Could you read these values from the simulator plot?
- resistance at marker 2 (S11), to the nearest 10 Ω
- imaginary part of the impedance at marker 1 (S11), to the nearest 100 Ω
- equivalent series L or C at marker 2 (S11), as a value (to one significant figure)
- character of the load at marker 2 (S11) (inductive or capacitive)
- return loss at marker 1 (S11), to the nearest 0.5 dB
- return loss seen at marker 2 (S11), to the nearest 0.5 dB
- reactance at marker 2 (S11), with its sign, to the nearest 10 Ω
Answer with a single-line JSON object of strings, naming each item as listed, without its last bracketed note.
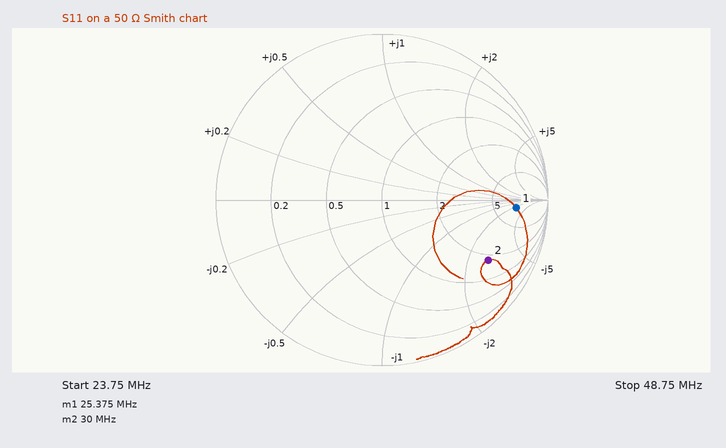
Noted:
{"resistance at marker 2 (S11), to the nearest 10 Ω": "90 Ω", "imaginary part of the impedance at marker 1 (S11), to the nearest 100 Ω": "-100 Ω", "equivalent series L or C at marker 2 (S11), as a value": "40 pF", "character of the load at marker 2 (S11)": "capacitive", "return loss at marker 1 (S11), to the nearest 0.5 dB": "2.0 dB", "return loss seen at marker 2 (S11), to the nearest 0.5 dB": "2.5 dB", "reactance at marker 2 (S11), with its sign, to the nearest 10 Ω": "-140 Ω"}
